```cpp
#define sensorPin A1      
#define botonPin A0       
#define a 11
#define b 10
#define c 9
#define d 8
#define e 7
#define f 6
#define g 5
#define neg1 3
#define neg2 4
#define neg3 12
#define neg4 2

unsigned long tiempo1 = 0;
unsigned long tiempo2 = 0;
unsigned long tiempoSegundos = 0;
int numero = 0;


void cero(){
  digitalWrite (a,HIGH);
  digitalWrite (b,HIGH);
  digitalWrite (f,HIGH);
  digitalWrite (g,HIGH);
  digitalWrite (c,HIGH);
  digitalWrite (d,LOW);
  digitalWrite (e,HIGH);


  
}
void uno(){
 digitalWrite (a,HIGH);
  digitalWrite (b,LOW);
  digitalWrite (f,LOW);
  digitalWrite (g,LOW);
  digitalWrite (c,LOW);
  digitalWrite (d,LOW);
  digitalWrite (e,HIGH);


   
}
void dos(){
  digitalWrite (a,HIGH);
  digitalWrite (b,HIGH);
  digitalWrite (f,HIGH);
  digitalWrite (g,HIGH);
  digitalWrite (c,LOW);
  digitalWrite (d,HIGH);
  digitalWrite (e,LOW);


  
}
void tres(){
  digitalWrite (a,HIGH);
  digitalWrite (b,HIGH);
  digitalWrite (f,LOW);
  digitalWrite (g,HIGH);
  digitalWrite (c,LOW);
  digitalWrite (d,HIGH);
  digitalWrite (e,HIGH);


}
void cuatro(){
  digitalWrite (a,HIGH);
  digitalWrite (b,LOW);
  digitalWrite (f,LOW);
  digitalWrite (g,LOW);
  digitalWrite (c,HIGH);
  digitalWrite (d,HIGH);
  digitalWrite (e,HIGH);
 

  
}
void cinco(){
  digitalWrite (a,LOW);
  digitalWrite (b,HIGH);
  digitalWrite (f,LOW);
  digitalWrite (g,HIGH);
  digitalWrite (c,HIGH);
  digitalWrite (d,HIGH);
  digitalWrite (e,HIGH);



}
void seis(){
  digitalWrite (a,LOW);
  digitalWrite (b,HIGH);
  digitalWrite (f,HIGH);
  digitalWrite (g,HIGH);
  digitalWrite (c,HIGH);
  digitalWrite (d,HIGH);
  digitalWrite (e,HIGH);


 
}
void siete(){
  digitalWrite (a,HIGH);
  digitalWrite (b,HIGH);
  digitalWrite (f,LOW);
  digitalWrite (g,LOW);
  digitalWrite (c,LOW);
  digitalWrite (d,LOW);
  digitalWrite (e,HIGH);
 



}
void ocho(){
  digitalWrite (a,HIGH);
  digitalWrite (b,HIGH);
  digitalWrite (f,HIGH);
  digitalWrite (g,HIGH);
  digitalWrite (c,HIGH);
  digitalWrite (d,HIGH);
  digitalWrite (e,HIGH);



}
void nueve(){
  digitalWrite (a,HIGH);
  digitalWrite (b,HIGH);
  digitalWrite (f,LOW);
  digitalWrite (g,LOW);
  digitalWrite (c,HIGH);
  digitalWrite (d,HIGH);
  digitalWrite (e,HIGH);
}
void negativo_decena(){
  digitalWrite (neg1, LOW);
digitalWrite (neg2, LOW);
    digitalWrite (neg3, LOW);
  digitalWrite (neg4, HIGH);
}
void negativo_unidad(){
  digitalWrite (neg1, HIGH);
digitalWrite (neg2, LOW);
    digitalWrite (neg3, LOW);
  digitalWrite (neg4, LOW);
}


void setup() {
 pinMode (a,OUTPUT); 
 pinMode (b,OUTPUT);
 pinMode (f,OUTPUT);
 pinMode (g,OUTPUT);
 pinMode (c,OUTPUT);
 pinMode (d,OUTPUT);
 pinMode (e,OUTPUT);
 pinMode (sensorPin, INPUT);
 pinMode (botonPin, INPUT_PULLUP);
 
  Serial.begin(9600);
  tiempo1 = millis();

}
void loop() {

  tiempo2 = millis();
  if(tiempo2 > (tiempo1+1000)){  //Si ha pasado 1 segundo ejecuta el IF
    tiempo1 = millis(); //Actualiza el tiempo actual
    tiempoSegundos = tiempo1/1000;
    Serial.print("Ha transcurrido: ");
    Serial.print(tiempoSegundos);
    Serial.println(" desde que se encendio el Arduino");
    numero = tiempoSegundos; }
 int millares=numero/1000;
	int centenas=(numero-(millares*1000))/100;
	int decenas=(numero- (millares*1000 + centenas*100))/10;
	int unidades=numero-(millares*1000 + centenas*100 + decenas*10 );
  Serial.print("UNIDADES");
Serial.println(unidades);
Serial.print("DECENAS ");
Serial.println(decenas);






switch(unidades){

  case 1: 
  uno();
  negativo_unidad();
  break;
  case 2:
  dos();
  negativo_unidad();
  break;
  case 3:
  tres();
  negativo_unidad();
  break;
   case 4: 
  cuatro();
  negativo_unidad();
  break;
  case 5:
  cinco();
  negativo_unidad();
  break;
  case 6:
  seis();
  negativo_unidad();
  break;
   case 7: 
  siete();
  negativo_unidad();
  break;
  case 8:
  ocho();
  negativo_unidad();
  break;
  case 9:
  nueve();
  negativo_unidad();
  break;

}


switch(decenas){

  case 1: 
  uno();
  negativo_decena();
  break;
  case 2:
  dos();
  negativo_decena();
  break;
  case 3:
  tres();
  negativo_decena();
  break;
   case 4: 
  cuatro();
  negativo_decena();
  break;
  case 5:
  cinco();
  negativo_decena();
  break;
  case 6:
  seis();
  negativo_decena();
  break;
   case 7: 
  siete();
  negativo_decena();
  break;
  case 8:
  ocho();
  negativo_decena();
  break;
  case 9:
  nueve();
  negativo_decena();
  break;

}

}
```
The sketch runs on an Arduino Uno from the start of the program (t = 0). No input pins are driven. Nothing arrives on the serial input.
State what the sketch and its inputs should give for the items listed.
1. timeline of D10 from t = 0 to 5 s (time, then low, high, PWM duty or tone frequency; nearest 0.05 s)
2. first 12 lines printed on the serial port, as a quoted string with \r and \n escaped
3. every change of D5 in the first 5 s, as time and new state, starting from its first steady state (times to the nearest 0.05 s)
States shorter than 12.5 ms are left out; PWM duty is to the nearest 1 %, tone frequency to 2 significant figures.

0 s low; 2.1 s high; 4.15 s low
"UNIDADES0\r\nDECENAS 0\r\nUNIDADES0\r\nDECENAS 0\r\nUNIDADES0\r\nDECENAS 0\r\nUNIDADES0\r\nDECENAS 0\r\nUNIDADES0\r\nDECENAS 0\r\nUNIDADES0\r\nDECENAS 0\r\n"
0 s low; 2.1 s high; 4.15 s low
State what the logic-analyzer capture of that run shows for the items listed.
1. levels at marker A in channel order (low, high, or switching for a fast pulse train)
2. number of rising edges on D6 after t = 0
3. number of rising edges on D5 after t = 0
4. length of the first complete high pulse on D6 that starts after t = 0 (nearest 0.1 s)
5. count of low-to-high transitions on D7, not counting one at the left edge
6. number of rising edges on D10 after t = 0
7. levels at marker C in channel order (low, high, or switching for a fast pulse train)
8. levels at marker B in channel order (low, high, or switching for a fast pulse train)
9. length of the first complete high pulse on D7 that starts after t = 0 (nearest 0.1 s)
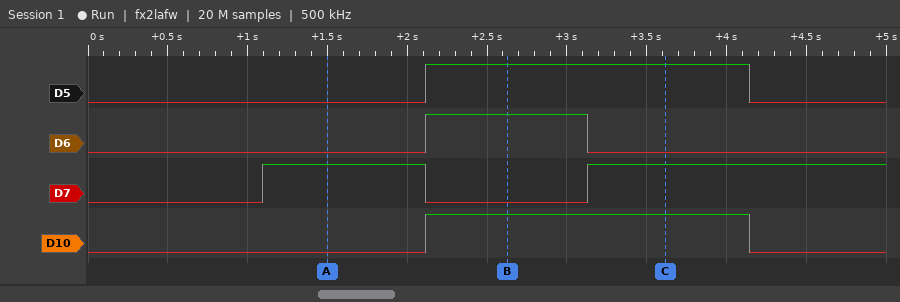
D5 low, D6 low, D7 high, D10 low
1
1
1.0 s
2
1
D5 high, D6 low, D7 high, D10 high
D5 high, D6 high, D7 low, D10 high
1.0 s
